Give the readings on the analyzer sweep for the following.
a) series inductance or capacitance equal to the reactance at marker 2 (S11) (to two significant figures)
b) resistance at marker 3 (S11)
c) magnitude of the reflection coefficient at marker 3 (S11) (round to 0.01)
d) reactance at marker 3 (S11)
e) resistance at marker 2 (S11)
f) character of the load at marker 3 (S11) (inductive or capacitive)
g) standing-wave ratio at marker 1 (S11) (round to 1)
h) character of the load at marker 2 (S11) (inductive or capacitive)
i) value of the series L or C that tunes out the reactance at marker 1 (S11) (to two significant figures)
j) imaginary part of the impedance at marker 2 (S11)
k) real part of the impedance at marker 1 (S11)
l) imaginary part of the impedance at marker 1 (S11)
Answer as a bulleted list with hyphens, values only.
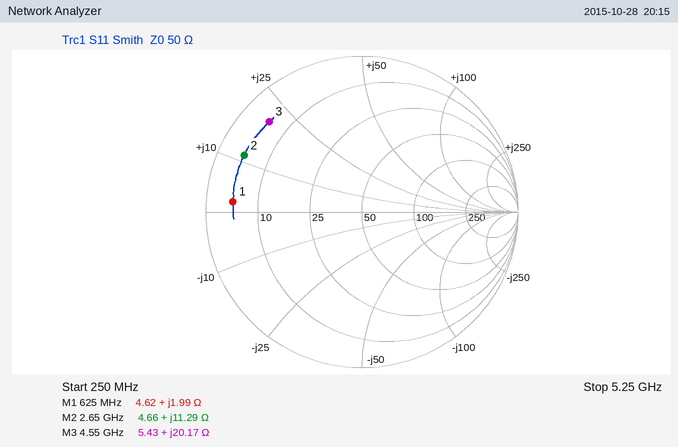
- 680 pH
- 5.43 Ω
- 0.83
- +20.17 Ω
- 4.66 Ω
- inductive
- 11
- inductive
- 130 pF
- +11.29 Ω
- 4.62 Ω
- +1.99 Ω
